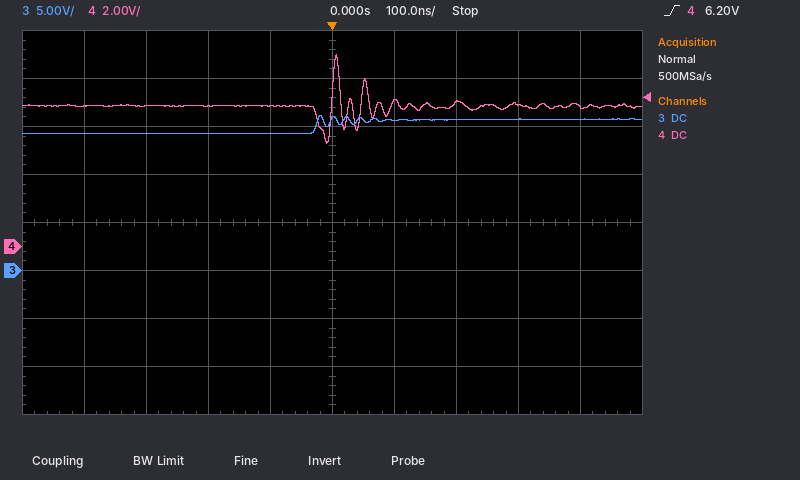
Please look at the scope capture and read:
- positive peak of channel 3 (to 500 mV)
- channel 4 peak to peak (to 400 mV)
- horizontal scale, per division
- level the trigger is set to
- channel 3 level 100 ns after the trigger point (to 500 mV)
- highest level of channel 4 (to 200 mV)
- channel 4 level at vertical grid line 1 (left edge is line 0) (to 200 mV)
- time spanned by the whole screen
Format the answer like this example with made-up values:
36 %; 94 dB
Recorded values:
16.0 V; 3.6 V; 100 ns; 6.20 V; 15.5 V; 8.0 V; 5.8 V; 1 µs
